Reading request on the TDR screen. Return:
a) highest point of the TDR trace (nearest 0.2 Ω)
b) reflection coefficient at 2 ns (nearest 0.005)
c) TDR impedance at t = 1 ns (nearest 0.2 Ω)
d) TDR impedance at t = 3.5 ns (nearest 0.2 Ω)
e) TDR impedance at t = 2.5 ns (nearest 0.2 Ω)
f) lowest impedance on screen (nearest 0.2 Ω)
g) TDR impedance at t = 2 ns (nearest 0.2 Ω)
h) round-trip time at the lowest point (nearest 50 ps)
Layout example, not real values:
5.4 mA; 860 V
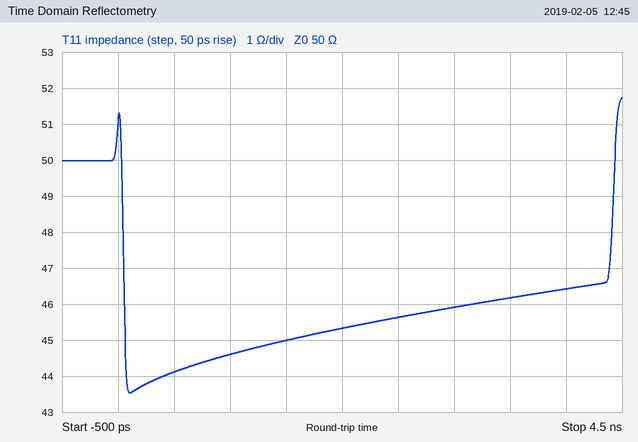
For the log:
51.8 Ω; -0.050; 44.6 Ω; 46.2 Ω; 45.6 Ω; 43.6 Ω; 45.4 Ω; 100 ps
